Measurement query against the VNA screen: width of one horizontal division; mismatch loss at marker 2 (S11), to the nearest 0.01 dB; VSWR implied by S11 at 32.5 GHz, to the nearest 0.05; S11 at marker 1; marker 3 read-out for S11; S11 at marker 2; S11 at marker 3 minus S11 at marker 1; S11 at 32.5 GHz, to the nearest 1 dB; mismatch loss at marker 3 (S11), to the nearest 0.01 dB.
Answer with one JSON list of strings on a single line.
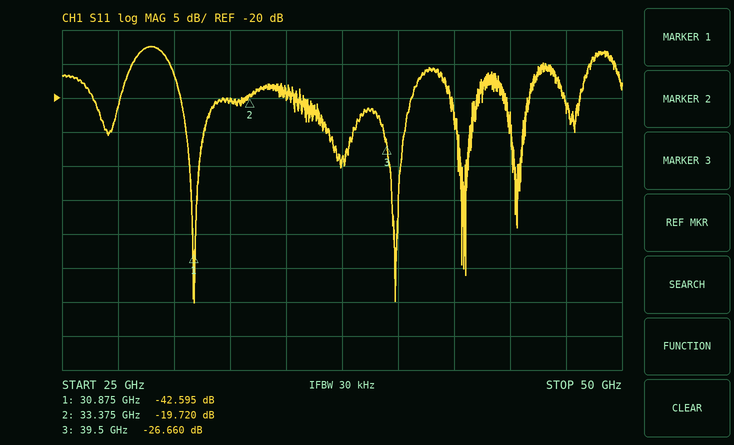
["2.5 GHz", "0.05 dB", "1.20", "-42.595 dB", "-26.660 dB", "-19.720 dB", "15.935 dB", "-20 dB", "0.01 dB"]
